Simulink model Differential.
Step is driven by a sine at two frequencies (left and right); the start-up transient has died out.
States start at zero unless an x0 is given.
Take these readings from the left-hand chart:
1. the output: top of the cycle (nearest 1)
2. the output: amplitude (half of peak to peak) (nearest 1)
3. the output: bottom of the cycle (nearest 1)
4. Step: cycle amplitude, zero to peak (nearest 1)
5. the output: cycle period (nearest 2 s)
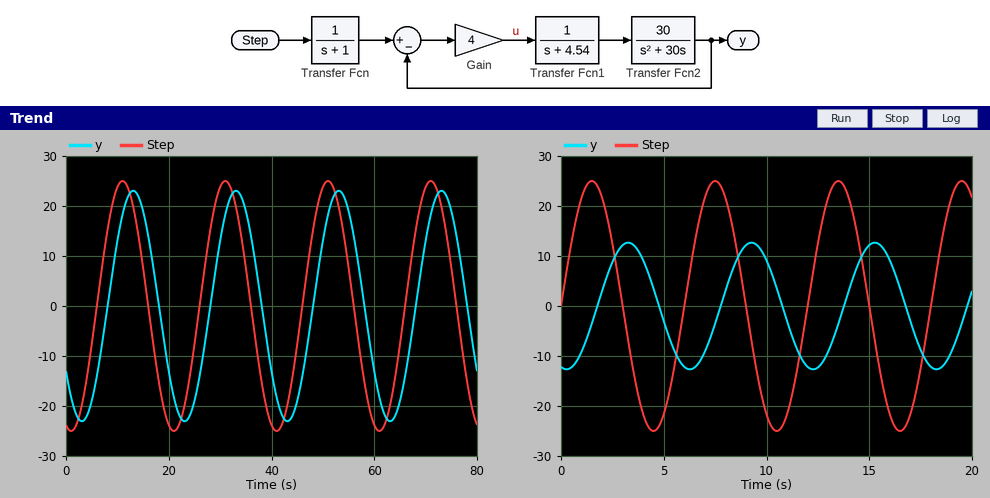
23
23
-23
25
20 s
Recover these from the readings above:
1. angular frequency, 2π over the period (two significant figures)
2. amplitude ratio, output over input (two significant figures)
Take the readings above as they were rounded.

0.31 rad/s
0.92
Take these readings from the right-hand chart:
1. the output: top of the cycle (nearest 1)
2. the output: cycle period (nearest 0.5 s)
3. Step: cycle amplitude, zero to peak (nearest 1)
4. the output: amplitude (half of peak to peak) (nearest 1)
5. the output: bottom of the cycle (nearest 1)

13
6.0 s
25
13
-13
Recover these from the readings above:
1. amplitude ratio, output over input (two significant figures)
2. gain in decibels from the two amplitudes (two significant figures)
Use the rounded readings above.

0.52
-5.7 dB
